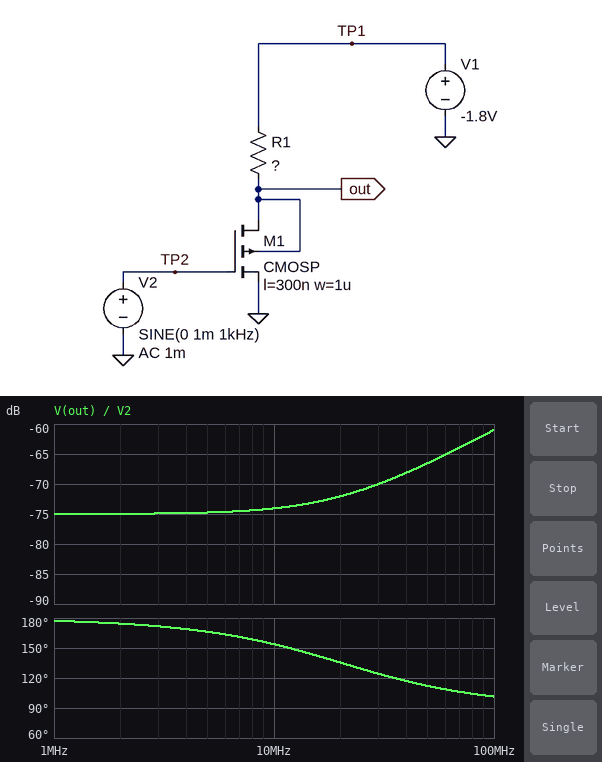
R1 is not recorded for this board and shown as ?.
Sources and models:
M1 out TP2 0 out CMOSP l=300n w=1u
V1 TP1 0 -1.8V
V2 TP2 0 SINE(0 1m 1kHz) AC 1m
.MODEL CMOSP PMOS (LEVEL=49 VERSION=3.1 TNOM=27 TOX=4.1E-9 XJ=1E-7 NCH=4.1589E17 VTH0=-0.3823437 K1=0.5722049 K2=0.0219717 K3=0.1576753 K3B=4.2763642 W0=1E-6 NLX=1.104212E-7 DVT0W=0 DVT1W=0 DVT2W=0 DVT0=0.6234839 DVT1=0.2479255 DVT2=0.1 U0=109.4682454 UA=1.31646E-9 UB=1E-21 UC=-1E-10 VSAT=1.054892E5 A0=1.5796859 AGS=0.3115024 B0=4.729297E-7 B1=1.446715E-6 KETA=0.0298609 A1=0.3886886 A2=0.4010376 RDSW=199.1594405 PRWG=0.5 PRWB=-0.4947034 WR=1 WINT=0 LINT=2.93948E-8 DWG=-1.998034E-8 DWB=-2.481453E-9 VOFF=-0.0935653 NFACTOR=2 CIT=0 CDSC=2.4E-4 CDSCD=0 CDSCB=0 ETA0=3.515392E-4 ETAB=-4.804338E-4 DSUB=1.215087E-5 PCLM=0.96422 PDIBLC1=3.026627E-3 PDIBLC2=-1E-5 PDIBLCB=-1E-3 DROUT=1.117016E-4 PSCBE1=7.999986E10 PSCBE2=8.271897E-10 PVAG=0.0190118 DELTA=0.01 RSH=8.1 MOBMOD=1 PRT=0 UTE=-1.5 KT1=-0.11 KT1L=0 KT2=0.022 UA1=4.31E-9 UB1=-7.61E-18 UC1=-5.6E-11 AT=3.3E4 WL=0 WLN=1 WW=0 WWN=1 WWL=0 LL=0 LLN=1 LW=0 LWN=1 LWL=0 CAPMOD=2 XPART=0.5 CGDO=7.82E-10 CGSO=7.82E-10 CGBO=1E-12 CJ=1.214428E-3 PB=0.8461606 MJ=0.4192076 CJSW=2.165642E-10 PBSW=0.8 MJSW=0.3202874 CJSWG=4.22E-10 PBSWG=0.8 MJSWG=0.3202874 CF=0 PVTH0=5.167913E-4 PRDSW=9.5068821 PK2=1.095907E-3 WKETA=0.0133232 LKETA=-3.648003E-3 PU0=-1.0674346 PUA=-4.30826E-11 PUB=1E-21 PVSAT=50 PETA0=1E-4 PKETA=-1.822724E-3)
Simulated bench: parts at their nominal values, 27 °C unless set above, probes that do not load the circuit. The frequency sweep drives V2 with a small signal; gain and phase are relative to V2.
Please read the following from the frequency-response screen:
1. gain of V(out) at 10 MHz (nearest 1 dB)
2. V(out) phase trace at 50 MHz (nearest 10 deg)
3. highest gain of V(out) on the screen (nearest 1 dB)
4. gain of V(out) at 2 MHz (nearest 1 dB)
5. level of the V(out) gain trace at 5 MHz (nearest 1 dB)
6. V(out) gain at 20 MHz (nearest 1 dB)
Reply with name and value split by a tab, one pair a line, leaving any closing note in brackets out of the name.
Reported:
gain of V(out) at 10 MHz	-74 dB
V(out) phase trace at 50 MHz	110 deg
highest gain of V(out) on the screen	-61 dB
gain of V(out) at 2 MHz	-75 dB
level of the V(out) gain trace at 5 MHz	-75 dB
V(out) gain at 20 MHz	-72 dB
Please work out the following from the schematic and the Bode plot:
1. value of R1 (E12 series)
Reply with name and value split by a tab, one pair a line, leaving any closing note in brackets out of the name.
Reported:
value of R1	820 Ω
